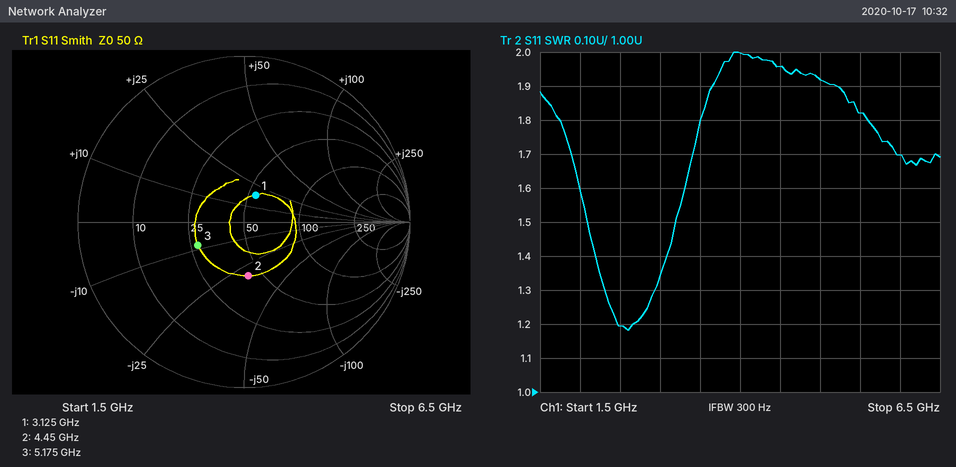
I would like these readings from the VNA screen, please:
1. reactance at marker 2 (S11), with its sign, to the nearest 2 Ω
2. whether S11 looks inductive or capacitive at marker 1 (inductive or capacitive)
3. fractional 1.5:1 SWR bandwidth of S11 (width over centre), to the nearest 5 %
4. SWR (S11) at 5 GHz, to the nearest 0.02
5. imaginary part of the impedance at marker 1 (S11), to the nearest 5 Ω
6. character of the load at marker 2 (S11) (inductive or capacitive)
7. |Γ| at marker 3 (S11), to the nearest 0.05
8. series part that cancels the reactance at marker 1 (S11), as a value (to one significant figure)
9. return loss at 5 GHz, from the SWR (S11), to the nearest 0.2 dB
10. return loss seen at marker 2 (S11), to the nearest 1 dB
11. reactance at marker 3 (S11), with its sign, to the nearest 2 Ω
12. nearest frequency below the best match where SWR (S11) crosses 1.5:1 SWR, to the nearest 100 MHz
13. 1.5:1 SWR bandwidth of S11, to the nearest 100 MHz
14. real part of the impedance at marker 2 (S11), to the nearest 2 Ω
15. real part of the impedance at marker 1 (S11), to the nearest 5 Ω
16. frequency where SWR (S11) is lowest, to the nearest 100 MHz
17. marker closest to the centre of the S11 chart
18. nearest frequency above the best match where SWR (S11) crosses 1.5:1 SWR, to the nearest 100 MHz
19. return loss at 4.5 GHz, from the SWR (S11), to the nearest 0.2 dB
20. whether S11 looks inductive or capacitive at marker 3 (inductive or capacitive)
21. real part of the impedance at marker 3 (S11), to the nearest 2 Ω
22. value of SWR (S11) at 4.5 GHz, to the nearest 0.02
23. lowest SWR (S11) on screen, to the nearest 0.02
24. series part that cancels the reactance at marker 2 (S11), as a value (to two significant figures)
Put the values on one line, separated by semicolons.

-30 Ω; inductive; 40 %; 1.92; +20 Ω; capacitive; 0.30; 3 pF; 10.0 dB; 10 dB; -8 Ω; 2.1 GHz; 1.1 GHz; 42 Ω; 55 Ω; 2.6 GHz; marker 1; 3.2 GHz; 9.8 dB; capacitive; 28 Ω; 1.96; 1.18; 1.1 nH
